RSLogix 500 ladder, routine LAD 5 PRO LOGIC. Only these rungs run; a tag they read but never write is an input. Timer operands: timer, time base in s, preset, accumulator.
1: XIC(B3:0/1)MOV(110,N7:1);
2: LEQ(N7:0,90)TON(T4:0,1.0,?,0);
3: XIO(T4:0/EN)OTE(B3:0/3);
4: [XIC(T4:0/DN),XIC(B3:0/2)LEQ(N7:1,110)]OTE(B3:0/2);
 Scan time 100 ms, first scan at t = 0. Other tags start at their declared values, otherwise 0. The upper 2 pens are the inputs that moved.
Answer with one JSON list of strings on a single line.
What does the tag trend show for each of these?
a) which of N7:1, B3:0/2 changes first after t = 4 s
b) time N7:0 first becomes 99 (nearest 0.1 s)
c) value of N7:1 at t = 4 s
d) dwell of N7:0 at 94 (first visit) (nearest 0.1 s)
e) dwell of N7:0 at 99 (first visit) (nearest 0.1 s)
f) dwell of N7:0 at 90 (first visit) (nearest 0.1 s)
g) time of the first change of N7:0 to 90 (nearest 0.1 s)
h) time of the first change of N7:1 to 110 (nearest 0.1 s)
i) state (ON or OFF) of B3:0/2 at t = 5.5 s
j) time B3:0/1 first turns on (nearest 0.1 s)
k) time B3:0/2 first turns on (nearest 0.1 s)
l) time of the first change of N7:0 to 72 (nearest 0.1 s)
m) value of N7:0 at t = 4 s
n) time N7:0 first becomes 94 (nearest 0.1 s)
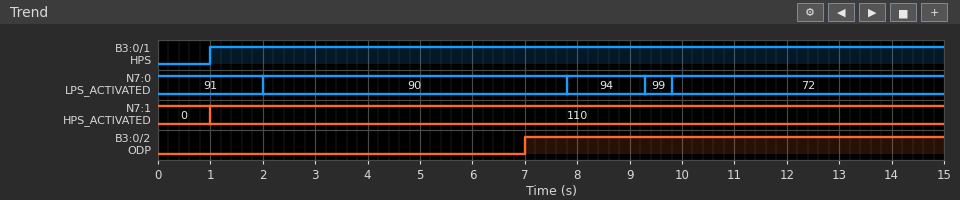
["B3:0/2", "9.3 s", "110", "1.5 s", "0.5 s", "5.8 s", "2.0 s", "1.0 s", "OFF", "1.0 s", "7.0 s", "9.8 s", "90", "7.8 s"]
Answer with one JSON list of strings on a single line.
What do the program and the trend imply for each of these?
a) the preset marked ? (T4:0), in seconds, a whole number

["5 s"]
